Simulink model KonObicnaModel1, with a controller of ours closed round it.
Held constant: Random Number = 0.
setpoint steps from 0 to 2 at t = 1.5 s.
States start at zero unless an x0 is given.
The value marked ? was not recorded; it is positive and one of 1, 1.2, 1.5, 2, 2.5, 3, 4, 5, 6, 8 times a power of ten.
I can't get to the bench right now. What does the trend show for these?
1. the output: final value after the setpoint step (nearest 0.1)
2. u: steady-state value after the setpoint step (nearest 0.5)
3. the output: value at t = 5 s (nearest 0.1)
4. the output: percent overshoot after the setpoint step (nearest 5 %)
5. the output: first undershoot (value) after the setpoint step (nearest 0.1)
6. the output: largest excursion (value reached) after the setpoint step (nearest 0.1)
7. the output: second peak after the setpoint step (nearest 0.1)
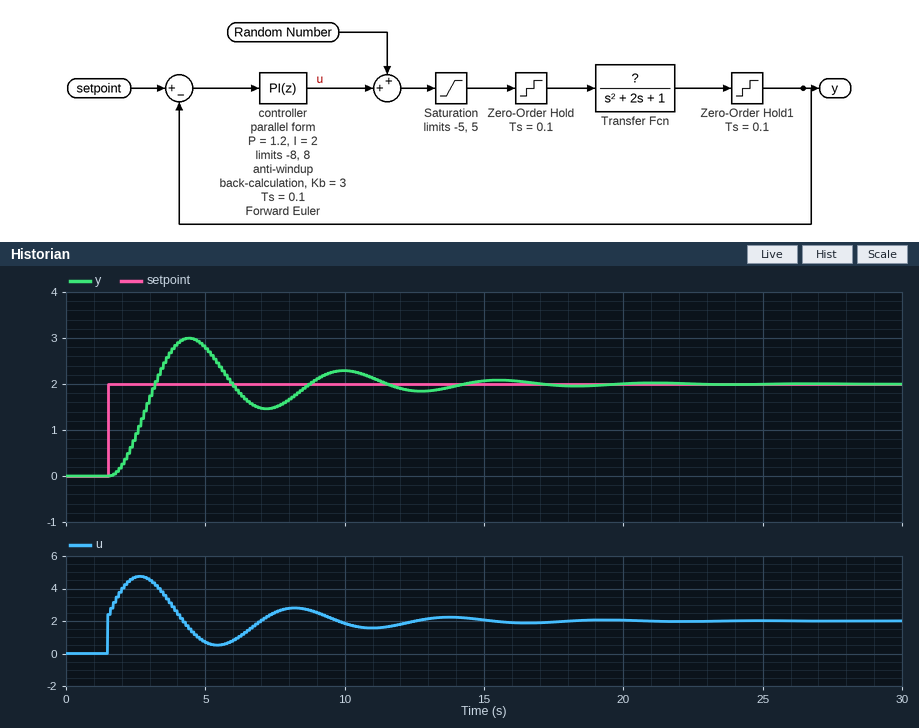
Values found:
2.0
2.0
2.8
50 %
1.5
3.0
2.3
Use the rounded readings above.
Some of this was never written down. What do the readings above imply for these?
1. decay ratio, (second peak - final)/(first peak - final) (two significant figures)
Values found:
0.30
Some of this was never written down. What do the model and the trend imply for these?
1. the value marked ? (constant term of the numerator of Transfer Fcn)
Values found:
1
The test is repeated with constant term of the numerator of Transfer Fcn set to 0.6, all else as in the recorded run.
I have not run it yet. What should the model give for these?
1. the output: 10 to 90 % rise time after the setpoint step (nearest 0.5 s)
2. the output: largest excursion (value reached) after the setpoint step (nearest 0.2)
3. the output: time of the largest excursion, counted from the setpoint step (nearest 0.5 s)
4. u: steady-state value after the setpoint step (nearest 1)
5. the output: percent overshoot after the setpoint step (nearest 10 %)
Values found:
1.5 s
2.6
4.5 s
3
30 %
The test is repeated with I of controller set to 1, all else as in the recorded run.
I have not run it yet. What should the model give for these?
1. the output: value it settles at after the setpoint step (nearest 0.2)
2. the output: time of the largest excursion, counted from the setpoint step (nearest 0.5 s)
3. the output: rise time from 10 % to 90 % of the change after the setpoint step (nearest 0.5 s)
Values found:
2.0
3.5 s
1.5 s
